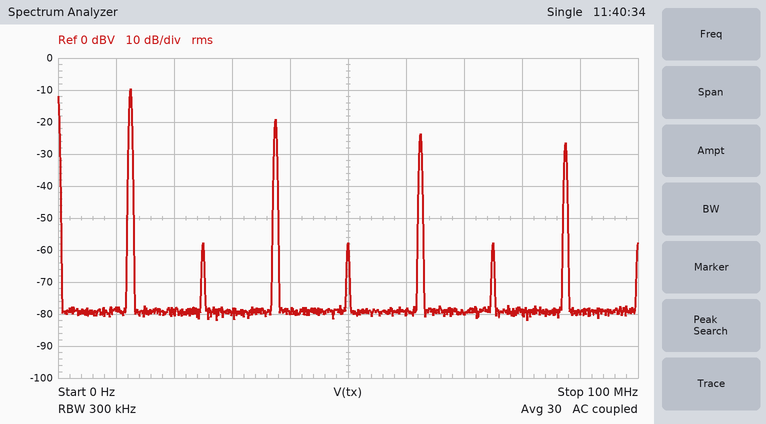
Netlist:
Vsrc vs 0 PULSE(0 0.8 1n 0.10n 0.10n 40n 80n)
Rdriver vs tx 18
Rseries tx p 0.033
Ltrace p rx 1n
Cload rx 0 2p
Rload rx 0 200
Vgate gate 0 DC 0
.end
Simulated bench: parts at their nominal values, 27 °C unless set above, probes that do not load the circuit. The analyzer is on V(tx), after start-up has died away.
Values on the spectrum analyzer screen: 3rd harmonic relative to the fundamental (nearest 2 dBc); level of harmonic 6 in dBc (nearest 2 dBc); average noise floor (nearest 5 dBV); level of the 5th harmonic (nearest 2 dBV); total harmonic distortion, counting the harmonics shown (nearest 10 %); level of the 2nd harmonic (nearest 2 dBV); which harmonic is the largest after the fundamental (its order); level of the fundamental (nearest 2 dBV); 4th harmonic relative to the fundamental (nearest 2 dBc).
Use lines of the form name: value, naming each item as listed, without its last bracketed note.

3rd harmonic relative to the fundamental: -10 dBc
level of harmonic 6 in dBc: -48 dBc
average noise floor: -80 dBV
level of the 5th harmonic: -24 dBV
total harmonic distortion, counting the harmonics shown: 40 %
level of the 2nd harmonic: -58 dBV
which harmonic is the largest after the fundamental: 3
level of the fundamental: -10 dBV
4th harmonic relative to the fundamental: -48 dBc
